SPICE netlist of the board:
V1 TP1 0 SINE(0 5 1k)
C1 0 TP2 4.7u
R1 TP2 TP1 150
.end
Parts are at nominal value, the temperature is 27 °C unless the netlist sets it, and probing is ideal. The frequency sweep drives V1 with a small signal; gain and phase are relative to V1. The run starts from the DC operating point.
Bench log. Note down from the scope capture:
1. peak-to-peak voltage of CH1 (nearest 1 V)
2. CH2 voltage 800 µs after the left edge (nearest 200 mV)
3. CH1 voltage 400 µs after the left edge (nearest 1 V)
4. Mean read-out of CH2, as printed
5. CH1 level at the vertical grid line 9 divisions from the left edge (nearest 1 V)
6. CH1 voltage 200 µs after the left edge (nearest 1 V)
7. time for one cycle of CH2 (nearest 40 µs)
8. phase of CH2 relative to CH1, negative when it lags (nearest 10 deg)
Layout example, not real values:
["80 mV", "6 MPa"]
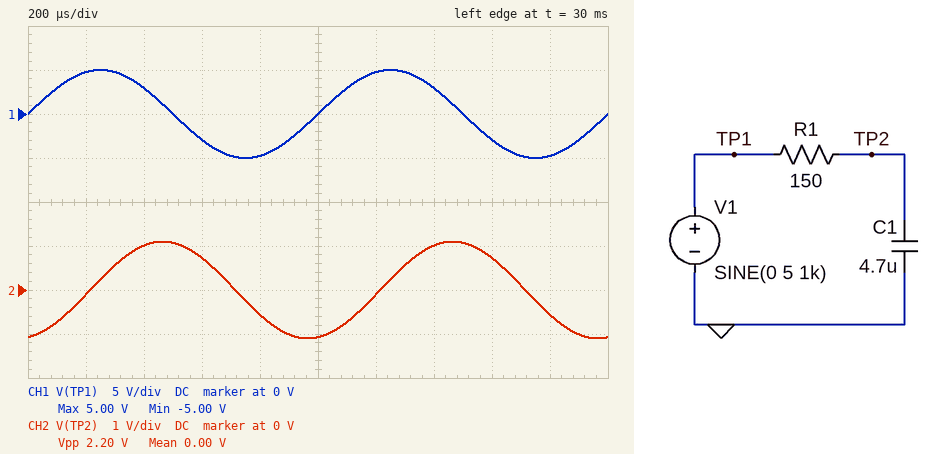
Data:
["10 V", "-600 mV", "3 V", "0.00 V", "-5 V", "5 V", "1.00 ms", "-80 deg"]
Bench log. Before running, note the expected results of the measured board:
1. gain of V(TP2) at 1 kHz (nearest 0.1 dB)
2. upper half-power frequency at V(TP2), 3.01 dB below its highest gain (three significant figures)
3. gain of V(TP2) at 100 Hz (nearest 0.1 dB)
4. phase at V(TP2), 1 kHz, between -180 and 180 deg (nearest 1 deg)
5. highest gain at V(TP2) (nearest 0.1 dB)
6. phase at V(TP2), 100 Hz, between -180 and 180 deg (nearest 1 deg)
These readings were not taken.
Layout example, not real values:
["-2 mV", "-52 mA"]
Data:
["-13.1 dB", "226 Hz", "-0.8 dB", "-77 deg", "0 dB", "-24 deg"]
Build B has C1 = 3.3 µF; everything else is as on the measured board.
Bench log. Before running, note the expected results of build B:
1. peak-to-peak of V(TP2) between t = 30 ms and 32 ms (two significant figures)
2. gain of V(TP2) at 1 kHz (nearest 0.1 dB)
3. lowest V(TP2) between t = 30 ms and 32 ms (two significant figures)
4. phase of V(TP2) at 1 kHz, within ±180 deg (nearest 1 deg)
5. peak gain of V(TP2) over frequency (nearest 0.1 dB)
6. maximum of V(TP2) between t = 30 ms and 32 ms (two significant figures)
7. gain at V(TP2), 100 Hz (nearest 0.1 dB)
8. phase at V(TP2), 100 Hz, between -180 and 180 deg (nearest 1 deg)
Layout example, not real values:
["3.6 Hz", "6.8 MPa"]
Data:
["3.1 V", "-10.3 dB", "-1.5 V", "-72 deg", "0 dB", "1.5 V", "-0.4 dB", "-17 deg"]
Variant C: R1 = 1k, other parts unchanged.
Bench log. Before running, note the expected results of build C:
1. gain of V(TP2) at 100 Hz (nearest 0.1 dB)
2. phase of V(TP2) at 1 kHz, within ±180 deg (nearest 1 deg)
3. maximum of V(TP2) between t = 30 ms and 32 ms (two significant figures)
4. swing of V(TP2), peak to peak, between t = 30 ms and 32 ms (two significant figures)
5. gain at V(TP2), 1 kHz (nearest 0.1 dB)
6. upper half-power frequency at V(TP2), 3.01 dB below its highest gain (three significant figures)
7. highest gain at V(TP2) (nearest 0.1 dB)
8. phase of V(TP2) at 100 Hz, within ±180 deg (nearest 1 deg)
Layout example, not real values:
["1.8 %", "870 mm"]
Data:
["-9.9 dB", "-88 deg", "170 mV", "340 mV", "-29.4 dB", "33.9 Hz", "0 dB", "-71 deg"]
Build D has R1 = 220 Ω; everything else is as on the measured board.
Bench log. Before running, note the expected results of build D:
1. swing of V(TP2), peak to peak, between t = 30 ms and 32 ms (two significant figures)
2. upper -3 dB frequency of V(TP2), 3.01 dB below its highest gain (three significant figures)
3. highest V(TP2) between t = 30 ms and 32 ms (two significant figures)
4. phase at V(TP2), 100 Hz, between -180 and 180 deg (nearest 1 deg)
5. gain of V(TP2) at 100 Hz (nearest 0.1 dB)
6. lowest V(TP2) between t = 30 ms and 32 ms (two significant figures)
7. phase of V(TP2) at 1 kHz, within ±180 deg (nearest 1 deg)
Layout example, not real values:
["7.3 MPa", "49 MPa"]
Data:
["1.5 V", "154 Hz", "760 mV", "-33 deg", "-1.5 dB", "-760 mV", "-81 deg"]
